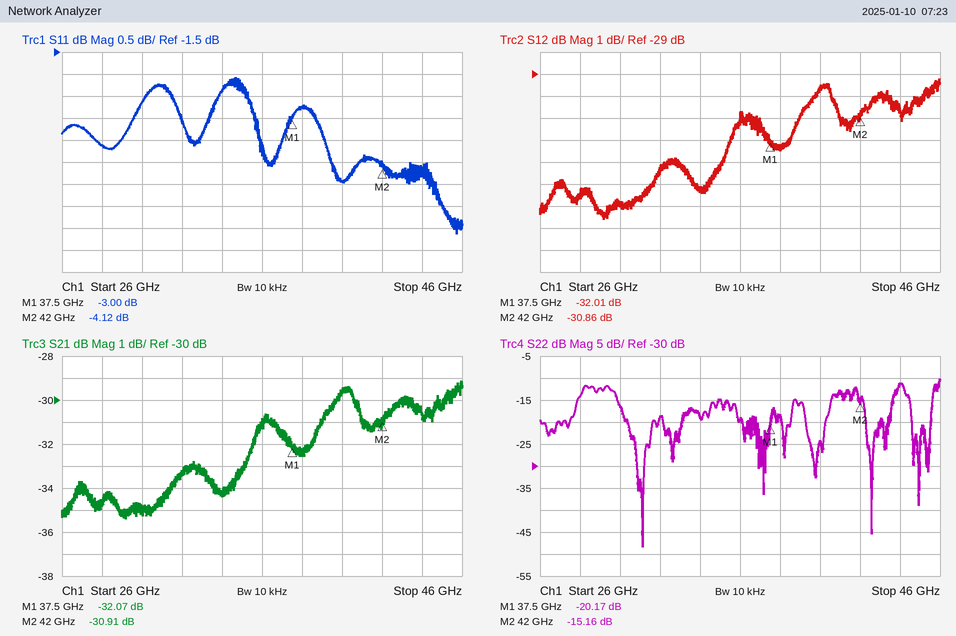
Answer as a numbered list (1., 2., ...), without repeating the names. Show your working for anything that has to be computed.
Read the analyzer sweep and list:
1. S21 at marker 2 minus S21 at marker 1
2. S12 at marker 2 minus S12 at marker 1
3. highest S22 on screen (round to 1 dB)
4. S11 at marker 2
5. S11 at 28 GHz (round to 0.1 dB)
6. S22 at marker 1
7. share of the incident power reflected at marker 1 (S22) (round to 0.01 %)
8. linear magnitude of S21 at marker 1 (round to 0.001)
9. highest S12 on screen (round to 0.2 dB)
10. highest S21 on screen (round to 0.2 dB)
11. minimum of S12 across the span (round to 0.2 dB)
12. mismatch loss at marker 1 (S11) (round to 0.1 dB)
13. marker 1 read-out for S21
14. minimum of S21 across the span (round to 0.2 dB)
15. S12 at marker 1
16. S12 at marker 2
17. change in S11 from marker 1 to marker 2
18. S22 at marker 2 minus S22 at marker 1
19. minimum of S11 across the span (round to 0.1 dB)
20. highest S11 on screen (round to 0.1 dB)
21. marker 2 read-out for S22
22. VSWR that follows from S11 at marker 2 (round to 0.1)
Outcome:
1. -30.91 − (-32.07) = 1.16 dB
2. -30.86 − (-32.01) = 1.15 dB
3. -10 dB
4. -4.12 dB
5. -3.6 dB
6. -20.17 dB
7. 10^(-20.17/10) ≈ 0.96 %
8. 10^(-32.07/20) ≈ 0.025
9. -29.2 dB
10. -29.2 dB
11. -35.6 dB
12. −10 log10(1 − 10^(-3/10)) ≈ 3.0 dB
13. -32.07 dB
14. -35.4 dB
15. -32.01 dB
16. -30.86 dB
17. -4.12 − (-3) = -1.12 dB
18. -15.16 − (-20.17) = 5.01 dB
19. -5.6 dB
20. -2.1 dB
21. -15.16 dB
22. (1 + 0.6223)/(1 − 0.6223) ≈ 4.3
